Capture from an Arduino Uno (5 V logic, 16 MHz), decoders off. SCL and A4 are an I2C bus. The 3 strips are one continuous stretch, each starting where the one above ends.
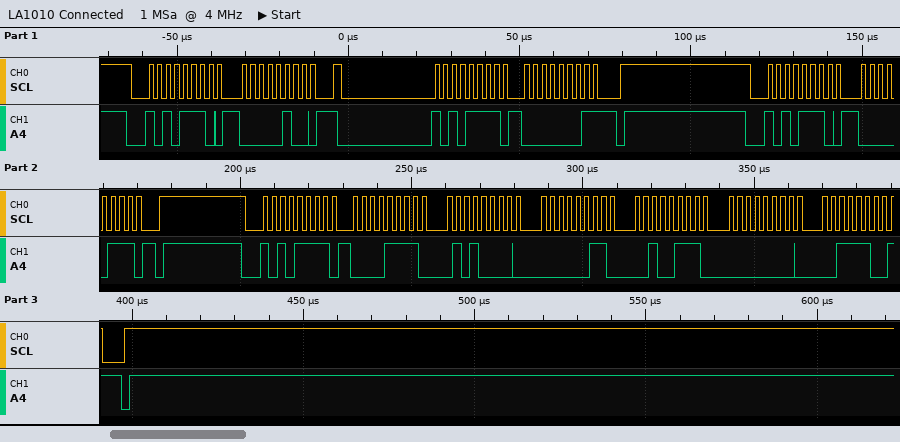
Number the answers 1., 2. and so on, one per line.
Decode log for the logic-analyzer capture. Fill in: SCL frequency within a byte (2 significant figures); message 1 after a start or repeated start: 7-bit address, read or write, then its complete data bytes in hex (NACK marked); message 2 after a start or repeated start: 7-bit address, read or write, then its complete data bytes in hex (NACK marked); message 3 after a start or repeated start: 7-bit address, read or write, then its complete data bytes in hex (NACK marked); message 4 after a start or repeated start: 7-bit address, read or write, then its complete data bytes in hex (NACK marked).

1. 400 kHz
2. 0x57 write: 04
3. 0x57 read: 01 NACK
4. 0x57 write: 07
5. 0x57 read: 0F 50 03 27 00 3C NACK
